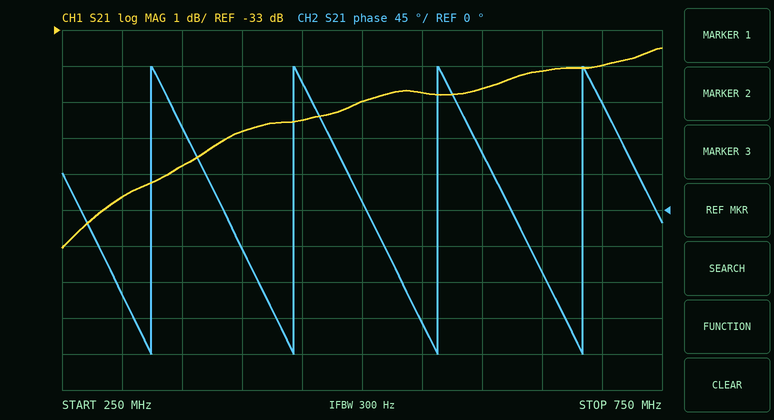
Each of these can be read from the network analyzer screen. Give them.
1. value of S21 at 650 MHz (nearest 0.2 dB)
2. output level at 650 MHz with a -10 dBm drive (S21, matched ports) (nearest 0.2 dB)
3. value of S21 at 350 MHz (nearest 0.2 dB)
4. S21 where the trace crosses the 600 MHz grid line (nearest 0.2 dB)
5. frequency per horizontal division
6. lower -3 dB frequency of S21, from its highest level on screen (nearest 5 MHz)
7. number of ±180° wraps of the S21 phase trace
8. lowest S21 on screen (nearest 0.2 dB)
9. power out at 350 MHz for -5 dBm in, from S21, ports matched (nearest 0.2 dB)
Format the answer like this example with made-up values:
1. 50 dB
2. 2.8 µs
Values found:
1. -34.2 dB
2. -44.2 dBm
3. -36.8 dB
4. -34.6 dB
5. 50 MHz
6. 365 MHz
7. 4
8. -39.0 dB
9. -41.8 dBm
